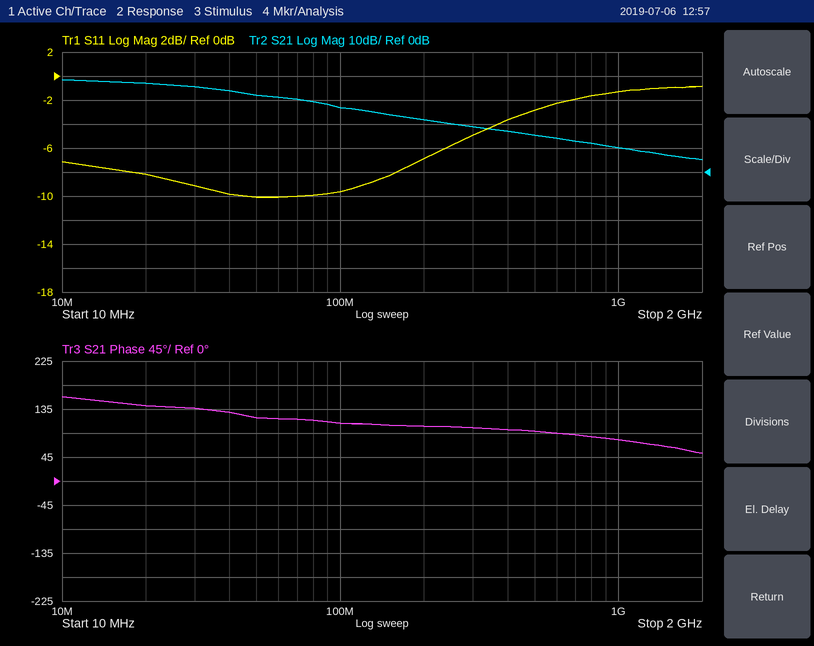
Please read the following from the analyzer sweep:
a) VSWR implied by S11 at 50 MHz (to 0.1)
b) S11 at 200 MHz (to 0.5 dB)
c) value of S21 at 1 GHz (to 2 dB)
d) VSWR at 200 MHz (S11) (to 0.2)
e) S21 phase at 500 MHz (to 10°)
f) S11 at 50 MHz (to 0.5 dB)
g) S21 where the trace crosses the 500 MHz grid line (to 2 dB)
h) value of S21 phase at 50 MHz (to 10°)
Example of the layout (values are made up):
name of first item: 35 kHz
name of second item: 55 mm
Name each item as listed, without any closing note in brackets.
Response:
VSWR implied by S11 at 50 MHz: 1.9
S11 at 200 MHz: -7.0 dB
value of S21 at 1 GHz: 10 dB
VSWR at 200 MHz (S11): 2.6
S21 phase at 500 MHz: 90°
S11 at 50 MHz: -10.0 dB
S21 where the trace crosses the 500 MHz grid line: 16 dB
value of S21 phase at 50 MHz: 120°
